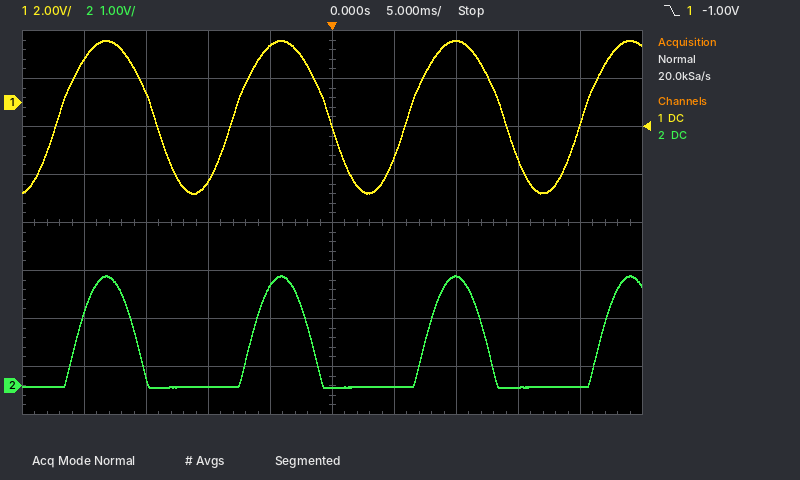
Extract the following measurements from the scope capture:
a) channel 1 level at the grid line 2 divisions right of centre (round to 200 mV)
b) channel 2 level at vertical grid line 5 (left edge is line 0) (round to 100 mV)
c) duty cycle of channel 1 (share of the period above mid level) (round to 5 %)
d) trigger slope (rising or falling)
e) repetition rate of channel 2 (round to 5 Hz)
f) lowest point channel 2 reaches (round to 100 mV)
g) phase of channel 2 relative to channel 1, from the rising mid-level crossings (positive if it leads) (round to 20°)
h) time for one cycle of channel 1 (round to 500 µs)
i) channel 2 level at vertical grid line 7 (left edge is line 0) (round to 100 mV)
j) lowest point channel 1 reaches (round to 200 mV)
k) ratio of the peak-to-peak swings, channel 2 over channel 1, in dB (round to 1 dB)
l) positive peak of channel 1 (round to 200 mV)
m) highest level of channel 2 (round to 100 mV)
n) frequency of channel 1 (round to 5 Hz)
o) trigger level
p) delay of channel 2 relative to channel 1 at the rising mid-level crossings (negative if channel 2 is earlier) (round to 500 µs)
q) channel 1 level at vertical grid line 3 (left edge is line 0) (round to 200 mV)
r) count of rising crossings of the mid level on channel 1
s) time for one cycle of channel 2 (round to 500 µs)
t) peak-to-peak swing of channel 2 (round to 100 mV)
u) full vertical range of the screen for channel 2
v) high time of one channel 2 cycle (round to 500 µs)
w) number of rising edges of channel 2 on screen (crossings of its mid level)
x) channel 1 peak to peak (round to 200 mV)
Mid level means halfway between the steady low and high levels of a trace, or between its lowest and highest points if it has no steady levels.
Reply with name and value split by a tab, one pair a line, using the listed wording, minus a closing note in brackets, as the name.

channel 1 level at the grid line 2 divisions right of centre	2.6 V
channel 2 level at vertical grid line 5 (left edge is line 0)	0.0 V
duty cycle of channel 1 (share of the period above mid level)	55 %
trigger slope	falling
repetition rate of channel 2	70 Hz
lowest point channel 2 reaches	0.0 V
phase of channel 2 relative to channel 1, from the rising mid-level crossings (positive if it leads)	-40°
time for one cycle of channel 1	14.0 ms
channel 2 level at vertical grid line 7 (left edge is line 0)	2.3 V
lowest point channel 1 reaches	-3.8 V
ratio of the peak-to-peak swings, channel 2 over channel 1, in dB	-9 dB
positive peak of channel 1	2.6 V
highest level of channel 2	2.3 V
frequency of channel 1	70 Hz
trigger level	-1.00 V
delay of channel 2 relative to channel 1 at the rising mid-level crossings (negative if channel 2 is earlier)	+1.5 ms
channel 1 level at vertical grid line 3 (left edge is line 0)	-3.2 V
count of rising crossings of the mid level on channel 1	4
time for one cycle of channel 2	14.0 ms
peak-to-peak swing of channel 2	2.3 V
full vertical range of the screen for channel 2	8 V
high time of one channel 2 cycle	4.5 ms
number of rising edges of channel 2 on screen	4
channel 1 peak to peak	6.4 V
